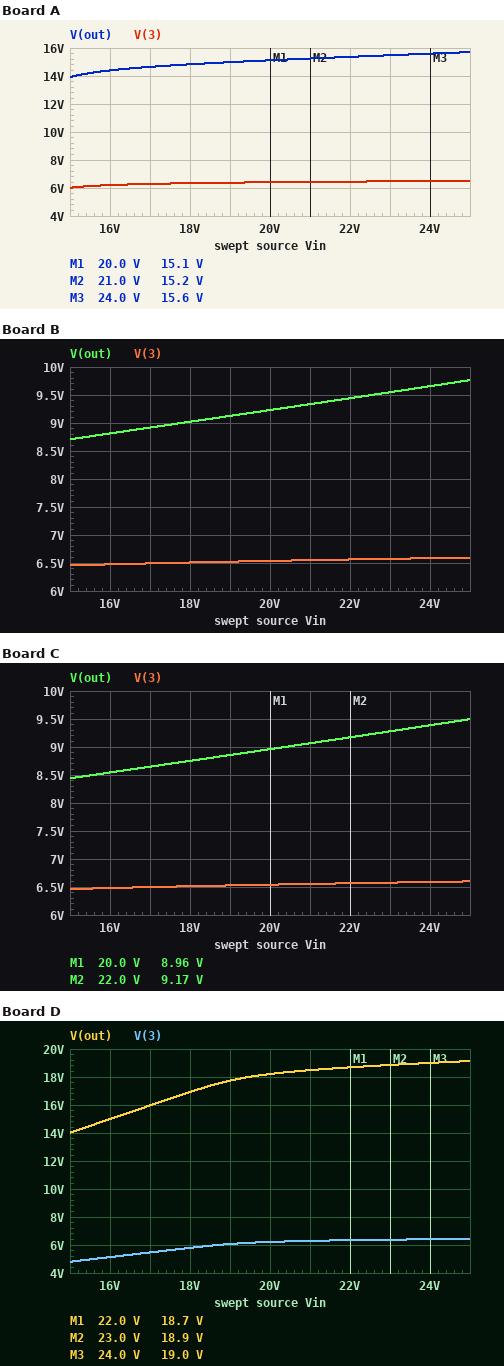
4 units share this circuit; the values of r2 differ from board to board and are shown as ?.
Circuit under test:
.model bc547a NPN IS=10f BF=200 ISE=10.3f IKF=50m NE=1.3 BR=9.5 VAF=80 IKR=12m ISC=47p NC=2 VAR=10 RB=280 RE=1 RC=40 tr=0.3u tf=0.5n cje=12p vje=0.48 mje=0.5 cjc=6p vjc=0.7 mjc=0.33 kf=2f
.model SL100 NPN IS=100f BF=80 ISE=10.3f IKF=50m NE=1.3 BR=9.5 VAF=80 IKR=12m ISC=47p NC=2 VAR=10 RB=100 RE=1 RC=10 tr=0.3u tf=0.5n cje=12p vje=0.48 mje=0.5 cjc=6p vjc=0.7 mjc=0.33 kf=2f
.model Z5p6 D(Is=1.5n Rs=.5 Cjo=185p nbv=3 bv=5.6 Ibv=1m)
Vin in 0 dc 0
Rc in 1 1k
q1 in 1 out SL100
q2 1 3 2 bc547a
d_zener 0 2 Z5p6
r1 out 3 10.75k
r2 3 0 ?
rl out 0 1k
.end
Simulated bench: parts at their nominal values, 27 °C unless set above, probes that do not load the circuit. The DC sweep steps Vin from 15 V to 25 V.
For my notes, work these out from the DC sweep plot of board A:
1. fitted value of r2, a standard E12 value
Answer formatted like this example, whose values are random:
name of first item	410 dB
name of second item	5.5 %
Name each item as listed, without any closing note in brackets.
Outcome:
fitted value of r2, a standard E12 value	8.2 kΩ
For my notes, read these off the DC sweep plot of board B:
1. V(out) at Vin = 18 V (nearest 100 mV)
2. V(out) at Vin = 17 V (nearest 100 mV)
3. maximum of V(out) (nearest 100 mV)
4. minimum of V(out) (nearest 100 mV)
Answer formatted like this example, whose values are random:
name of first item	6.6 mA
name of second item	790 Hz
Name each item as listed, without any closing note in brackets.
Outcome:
V(out) at Vin = 18 V	9.0 V
V(out) at Vin = 17 V	8.9 V
maximum of V(out)	9.8 V
minimum of V(out)	8.7 V
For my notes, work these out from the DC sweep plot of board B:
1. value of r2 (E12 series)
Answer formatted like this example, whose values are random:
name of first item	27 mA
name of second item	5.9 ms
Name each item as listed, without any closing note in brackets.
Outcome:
value of r2	39 kΩ
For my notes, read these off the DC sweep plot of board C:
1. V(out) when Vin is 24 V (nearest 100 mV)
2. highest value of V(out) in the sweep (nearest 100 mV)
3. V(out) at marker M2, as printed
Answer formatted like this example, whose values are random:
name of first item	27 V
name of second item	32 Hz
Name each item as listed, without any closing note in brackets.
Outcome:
V(out) when Vin is 24 V	9.4 V
highest value of V(out) in the sweep	9.5 V
V(out) at marker M2, as printed	9.17 V
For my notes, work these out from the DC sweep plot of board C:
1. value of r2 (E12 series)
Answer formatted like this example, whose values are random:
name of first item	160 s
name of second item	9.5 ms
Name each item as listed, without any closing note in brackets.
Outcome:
value of r2	47 kΩ
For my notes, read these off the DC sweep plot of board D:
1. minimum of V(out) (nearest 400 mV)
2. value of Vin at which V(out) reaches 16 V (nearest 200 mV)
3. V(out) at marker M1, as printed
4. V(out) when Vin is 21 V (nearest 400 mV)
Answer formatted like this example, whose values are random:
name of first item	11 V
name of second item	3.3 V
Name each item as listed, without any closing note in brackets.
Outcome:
minimum of V(out)	14.0 V
value of Vin at which V(out) reaches 16 V	17.0 V
V(out) at marker M1, as printed	18.7 V
V(out) when Vin is 21 V	18.4 V
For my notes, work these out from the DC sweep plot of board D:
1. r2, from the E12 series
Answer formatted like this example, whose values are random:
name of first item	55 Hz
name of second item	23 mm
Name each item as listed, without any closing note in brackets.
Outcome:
r2, from the E12 series	5.6 kΩ
